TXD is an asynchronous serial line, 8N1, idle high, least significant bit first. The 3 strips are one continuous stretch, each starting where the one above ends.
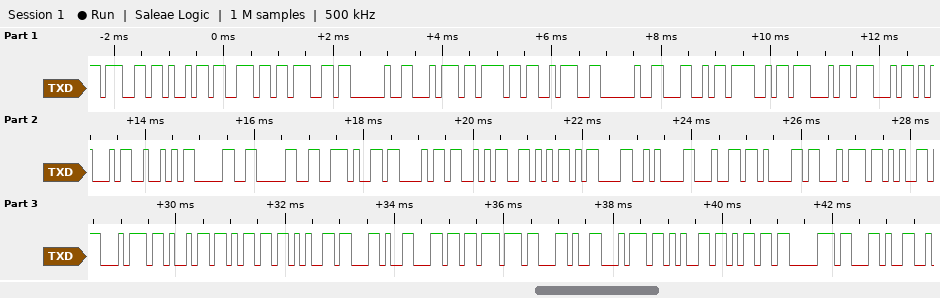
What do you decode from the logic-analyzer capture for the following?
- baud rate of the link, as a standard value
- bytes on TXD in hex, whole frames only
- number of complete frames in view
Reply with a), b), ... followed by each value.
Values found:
a) 9600 baud
b) 67 69 6E 67 20 74 6F 3A 20 4C 4F 47 47 45 52 30 30 2E 43 53 56 0D 0A 64 61 74 65 74 69 6D 65 2C 6C 77 2C 74 65 6D 70 2C
c) 40
